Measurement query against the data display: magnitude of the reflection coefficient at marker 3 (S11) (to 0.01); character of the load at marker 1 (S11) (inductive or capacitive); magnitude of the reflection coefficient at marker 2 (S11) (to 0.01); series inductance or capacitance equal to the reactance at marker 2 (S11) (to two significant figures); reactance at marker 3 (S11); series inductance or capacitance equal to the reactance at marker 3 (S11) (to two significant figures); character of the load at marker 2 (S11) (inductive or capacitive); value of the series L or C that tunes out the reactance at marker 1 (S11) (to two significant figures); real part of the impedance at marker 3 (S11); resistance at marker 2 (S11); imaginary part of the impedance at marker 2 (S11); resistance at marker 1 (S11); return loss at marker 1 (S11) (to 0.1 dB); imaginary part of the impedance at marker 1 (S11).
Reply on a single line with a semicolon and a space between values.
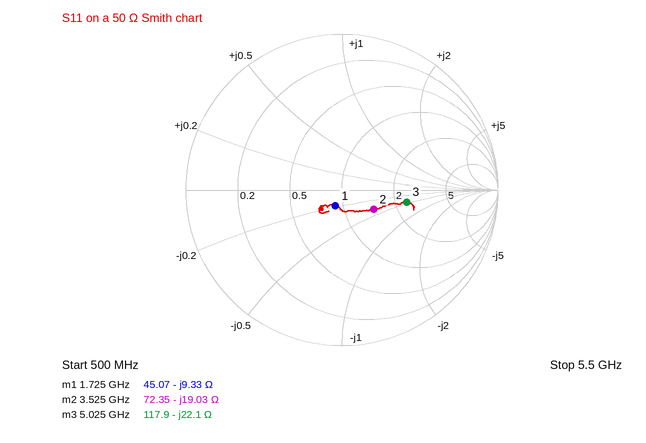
0.42; capacitive; 0.24; 2.4 pF; -22.1 Ω; 1.4 pF; capacitive; 860 pH; 117.9 Ω; 72.35 Ω; -19.03 Ω; 45.07 Ω; 19.1 dB; -9.33 Ω
